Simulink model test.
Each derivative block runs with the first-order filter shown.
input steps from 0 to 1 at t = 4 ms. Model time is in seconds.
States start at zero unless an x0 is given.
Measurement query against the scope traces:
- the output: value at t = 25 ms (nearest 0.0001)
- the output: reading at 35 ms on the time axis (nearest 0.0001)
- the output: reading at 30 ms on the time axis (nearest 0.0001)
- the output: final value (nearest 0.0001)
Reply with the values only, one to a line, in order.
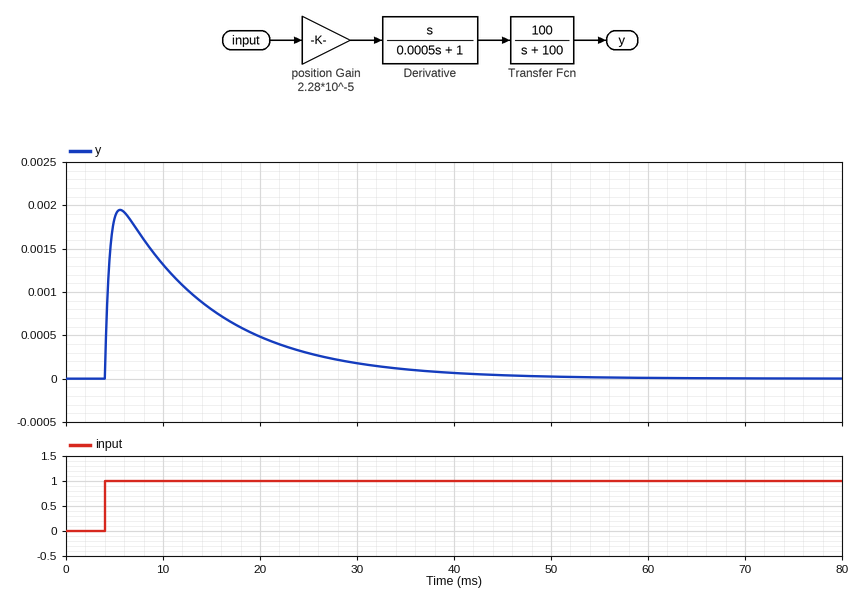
0.0003
0.0001
0.0002
0.0000
